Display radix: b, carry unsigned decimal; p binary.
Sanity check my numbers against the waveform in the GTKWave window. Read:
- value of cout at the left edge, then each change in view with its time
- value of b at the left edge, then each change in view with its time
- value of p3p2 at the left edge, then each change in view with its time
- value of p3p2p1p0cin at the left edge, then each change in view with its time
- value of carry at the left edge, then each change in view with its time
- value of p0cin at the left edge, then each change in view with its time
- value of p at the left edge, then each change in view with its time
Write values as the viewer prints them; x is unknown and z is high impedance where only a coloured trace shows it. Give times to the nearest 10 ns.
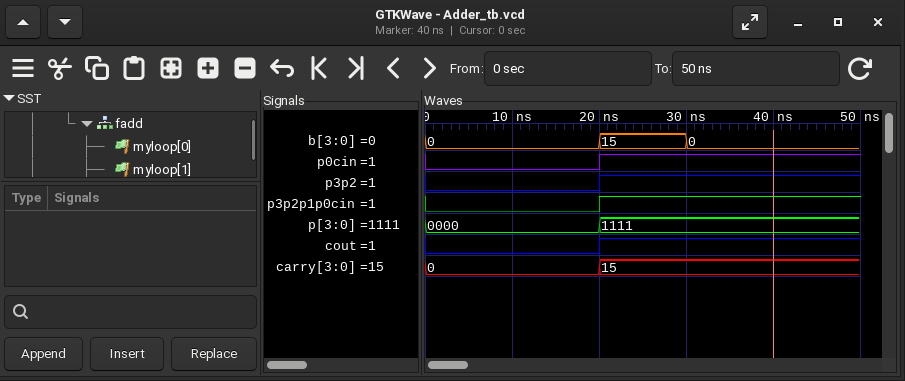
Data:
0, 1 at 20 ns
0, 15 at 20 ns, 0 at 30 ns
0, 1 at 20 ns
0, 1 at 20 ns
0, 15 at 20 ns
0, 1 at 20 ns
0000, 1111 at 20 ns
